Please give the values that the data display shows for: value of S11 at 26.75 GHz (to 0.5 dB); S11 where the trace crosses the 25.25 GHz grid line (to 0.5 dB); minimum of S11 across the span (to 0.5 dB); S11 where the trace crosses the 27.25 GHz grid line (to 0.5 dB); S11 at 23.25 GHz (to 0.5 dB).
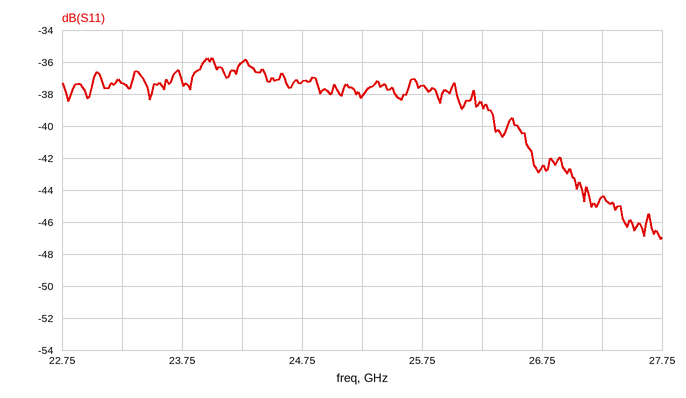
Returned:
-42.5 dB
-38.0 dB
-47.0 dB
-44.5 dB
-37.5 dB
